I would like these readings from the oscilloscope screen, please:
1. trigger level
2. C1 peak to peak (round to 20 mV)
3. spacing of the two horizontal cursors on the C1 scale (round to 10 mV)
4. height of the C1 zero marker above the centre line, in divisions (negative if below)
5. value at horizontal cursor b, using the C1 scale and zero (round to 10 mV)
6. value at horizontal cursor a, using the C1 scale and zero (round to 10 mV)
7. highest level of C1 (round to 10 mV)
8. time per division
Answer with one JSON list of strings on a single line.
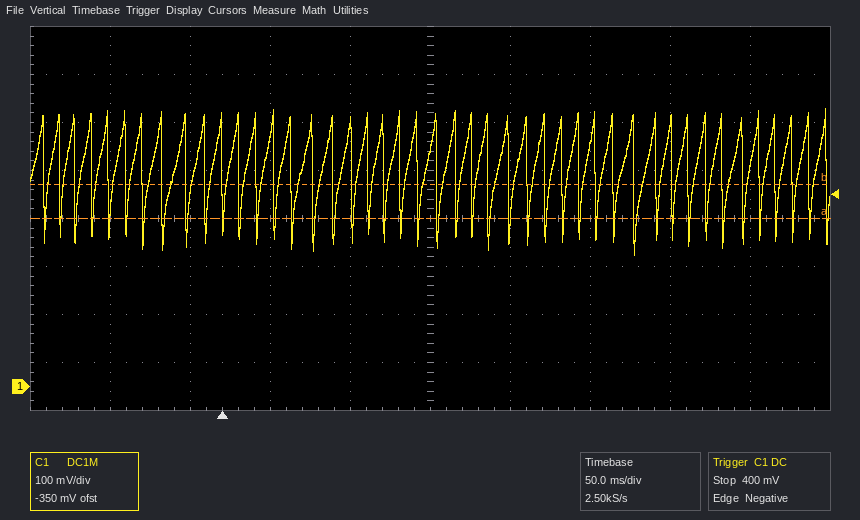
["400 mV", "300 mV", "70 mV", "-3.5 div", "420 mV", "350 mV", "580 mV", "50 ms"]
